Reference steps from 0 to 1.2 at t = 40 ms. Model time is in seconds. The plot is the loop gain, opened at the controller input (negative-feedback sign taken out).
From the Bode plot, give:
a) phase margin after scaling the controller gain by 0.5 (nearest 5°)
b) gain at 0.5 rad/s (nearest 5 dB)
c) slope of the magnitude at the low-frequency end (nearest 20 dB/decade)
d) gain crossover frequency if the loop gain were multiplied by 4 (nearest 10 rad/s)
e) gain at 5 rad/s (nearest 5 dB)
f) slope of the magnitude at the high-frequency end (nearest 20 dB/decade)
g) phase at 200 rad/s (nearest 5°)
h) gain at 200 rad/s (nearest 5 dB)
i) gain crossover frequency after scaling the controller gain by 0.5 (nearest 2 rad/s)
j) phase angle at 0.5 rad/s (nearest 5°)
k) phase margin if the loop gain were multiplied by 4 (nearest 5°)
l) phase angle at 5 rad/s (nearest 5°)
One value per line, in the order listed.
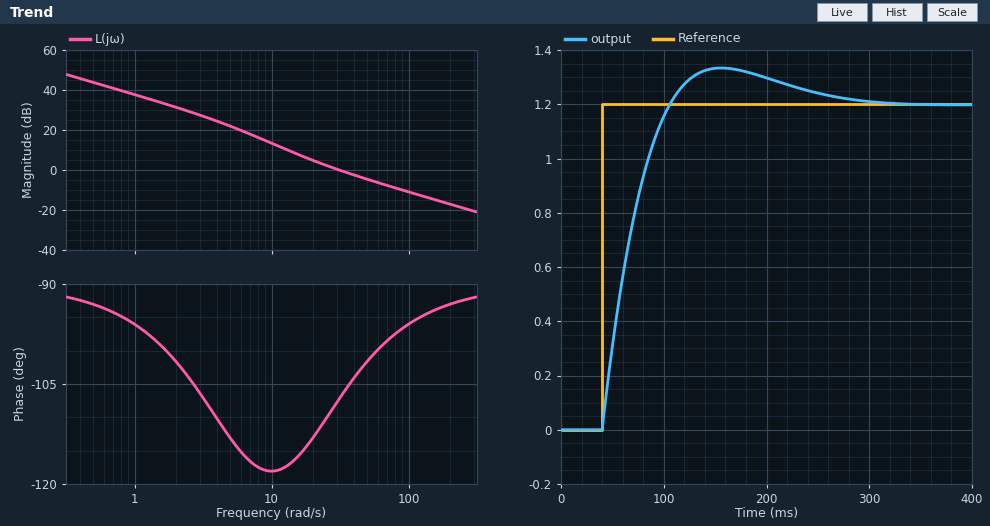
65°
45 dB
-20 dB/decade
110 rad/s
20 dB
-20 dB/decade
-95°
-15 dB
18 rad/s
-95°
85°
-115°
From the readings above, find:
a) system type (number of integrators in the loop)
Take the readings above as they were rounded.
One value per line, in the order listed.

1
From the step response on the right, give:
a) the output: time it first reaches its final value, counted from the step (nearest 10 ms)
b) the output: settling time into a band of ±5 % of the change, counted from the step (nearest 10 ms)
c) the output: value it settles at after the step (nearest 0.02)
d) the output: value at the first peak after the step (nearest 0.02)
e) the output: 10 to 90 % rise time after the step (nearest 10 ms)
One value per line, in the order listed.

70 ms
190 ms
1.20
1.34
50 ms
